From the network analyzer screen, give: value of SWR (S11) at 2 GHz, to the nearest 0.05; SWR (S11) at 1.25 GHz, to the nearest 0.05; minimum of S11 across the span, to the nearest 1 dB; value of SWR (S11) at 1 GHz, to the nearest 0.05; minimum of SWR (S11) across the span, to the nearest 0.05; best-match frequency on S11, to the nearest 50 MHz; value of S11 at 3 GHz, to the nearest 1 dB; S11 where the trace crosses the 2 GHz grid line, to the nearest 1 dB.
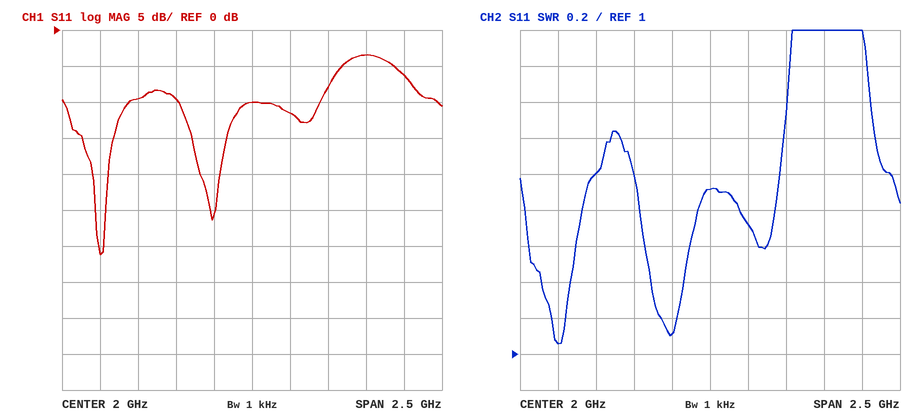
1.90
2.00
-31 dB
1.05
1.05
1.00 GHz
-6 dB
-10 dB
